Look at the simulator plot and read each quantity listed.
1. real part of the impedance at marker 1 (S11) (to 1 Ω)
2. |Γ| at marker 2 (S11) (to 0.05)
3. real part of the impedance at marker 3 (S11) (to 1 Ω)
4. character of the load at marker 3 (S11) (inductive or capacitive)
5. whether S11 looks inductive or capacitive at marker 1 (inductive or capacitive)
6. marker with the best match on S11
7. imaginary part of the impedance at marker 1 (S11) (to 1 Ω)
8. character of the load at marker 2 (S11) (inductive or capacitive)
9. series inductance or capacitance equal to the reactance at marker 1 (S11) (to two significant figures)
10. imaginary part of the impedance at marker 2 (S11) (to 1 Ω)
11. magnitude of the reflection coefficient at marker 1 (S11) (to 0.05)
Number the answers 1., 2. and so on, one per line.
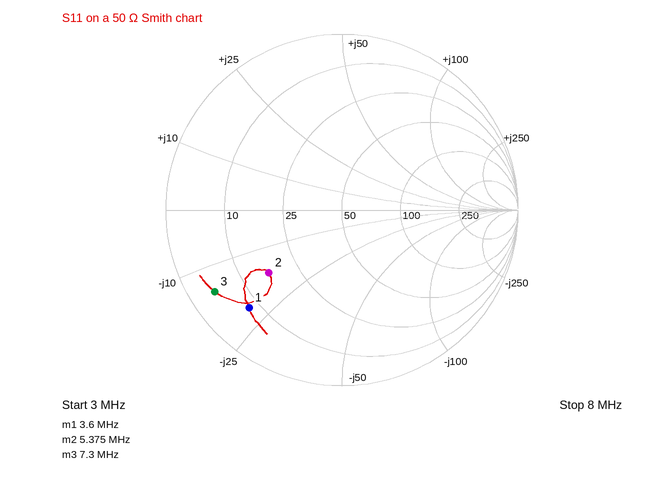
1. 8 Ω
2. 0.55
3. 4 Ω
4. capacitive
5. capacitive
6. marker 2
7. -21 Ω
8. capacitive
9. 2.1 nF
10. -17 Ω
11. 0.75
